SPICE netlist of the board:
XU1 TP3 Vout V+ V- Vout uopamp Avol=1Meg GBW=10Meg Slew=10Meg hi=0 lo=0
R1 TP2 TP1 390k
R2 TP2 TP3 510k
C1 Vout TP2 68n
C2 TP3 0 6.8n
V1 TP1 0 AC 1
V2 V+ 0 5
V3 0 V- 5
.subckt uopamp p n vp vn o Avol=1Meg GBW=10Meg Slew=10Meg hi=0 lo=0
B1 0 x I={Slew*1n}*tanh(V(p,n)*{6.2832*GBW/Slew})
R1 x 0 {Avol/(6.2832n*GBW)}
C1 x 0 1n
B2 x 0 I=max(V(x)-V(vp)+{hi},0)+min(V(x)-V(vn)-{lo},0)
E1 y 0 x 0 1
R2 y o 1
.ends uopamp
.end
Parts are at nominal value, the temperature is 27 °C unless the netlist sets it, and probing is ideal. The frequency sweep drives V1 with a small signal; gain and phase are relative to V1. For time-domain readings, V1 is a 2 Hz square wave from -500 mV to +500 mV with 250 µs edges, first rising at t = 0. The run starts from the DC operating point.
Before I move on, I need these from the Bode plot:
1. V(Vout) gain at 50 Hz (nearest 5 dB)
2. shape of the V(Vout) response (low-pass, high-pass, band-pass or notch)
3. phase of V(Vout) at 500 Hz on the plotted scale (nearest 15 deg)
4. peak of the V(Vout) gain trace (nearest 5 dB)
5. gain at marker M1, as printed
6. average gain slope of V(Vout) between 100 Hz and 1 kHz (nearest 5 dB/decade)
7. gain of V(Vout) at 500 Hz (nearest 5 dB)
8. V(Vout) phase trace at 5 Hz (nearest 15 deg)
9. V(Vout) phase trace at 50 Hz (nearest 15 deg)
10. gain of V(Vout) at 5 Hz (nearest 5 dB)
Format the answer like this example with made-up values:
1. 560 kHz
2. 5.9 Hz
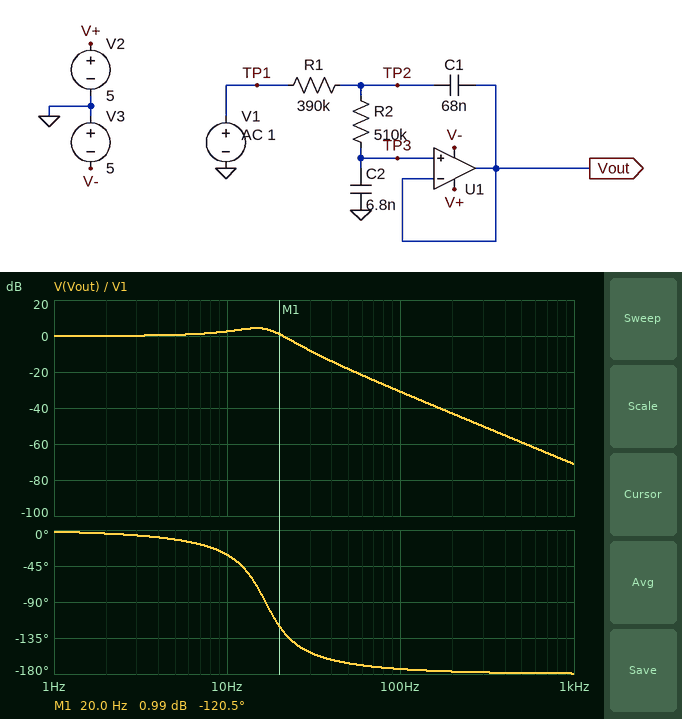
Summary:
1. -20 dB
2. low-pass
3. -180 deg
4. 5 dB
5. 0.99 dB
6. -40 dB/decade
7. -60 dB
8. -15 deg
9. -165 deg
10. 0 dB
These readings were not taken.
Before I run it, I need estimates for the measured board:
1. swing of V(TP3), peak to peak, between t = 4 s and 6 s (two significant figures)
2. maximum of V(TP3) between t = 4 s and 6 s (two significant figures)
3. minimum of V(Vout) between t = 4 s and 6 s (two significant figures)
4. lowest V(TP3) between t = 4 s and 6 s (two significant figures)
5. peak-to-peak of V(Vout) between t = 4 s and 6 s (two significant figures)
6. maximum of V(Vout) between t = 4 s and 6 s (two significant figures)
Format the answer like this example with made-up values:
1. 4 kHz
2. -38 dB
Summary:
1. 1.7 V
2. 850 mV
3. -850 mV
4. -850 mV
5. 1.7 V
6. 850 mV
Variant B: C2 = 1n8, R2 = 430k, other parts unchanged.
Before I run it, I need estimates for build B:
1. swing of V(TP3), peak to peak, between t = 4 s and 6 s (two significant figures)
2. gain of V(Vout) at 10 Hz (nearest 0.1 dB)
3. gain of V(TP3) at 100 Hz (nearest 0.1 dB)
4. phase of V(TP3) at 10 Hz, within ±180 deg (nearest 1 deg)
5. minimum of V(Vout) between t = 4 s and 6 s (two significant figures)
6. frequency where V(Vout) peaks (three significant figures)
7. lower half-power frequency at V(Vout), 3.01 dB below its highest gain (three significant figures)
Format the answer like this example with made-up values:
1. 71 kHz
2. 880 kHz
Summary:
1. 2.2 V
2. 0.7 dB
3. -17.1 dB
4. -6 deg
5. -1.1 V
6. 34.2 Hz
7. 27.8 Hz
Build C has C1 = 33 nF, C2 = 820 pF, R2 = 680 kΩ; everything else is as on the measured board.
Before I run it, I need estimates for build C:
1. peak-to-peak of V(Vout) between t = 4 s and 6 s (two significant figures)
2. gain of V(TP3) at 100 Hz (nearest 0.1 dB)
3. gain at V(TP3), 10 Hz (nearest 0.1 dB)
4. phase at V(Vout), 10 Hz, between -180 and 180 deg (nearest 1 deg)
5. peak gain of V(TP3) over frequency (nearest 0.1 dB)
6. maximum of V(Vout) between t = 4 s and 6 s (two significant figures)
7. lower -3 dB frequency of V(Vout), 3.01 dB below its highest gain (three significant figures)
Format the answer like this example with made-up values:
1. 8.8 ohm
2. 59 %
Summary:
1. 2.2 V
2. -5.6 dB
3. 0.2 dB
4. -3 deg
5. 9.8 dB
6. 1.1 V
7. 46.9 Hz
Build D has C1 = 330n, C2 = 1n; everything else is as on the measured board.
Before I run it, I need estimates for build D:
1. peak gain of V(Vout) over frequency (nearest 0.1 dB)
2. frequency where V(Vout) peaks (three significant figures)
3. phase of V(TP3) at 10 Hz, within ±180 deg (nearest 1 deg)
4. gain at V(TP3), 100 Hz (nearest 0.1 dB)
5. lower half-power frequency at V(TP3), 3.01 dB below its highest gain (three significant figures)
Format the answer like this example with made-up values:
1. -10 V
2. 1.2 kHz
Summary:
1. 19.1 dB
2. 19.6 Hz
3. -4 deg
4. -27.9 dB
5. 18.5 Hz
